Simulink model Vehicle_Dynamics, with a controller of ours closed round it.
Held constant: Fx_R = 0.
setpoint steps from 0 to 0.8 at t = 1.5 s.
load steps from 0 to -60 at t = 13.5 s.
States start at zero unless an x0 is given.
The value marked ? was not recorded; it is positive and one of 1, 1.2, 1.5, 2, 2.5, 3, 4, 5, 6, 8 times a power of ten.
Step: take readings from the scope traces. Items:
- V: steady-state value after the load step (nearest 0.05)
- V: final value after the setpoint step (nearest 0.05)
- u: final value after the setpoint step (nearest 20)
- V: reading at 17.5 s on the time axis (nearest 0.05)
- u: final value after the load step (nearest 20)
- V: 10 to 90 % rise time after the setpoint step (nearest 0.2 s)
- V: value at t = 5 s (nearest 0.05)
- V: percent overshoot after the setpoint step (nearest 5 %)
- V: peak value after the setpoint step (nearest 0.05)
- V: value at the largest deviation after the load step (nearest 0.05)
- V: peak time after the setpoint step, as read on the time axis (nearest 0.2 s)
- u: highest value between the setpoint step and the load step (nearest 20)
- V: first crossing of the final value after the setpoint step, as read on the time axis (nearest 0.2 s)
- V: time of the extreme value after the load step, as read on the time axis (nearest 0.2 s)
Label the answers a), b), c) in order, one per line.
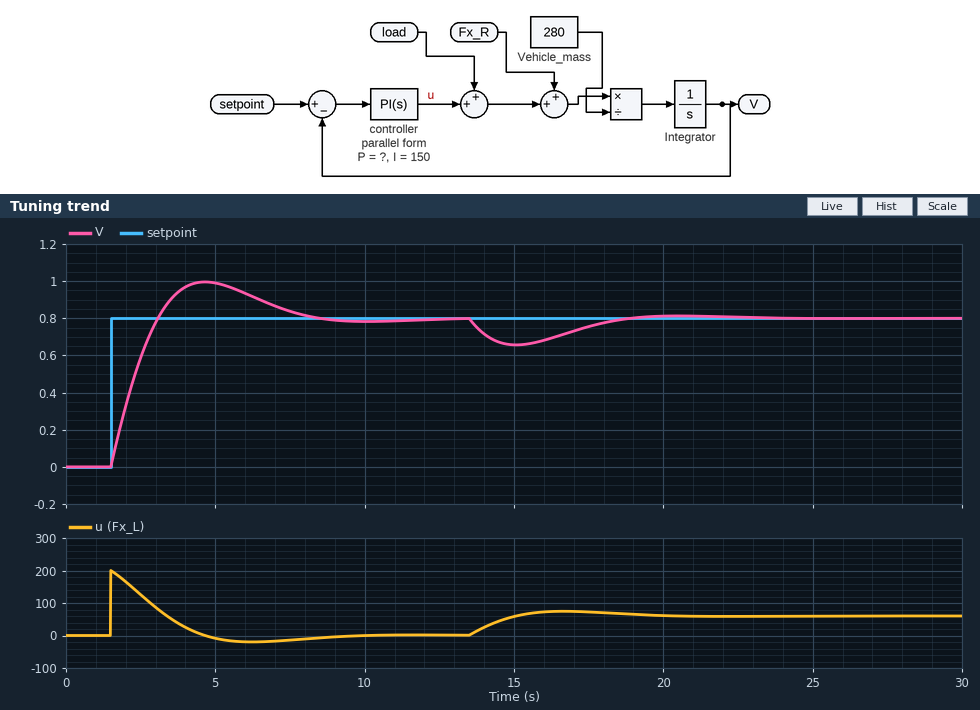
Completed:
a) 0.80
b) 0.80
c) 0
d) 0.75
e) 60
f) 1.2 s
g) 1.00
h) 25 %
i) 1.00
j) 0.65
k) 4.6 s
l) 200
m) 3.0 s
n) 15.0 s
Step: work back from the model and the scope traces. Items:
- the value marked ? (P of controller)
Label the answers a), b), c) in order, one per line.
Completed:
a) 250
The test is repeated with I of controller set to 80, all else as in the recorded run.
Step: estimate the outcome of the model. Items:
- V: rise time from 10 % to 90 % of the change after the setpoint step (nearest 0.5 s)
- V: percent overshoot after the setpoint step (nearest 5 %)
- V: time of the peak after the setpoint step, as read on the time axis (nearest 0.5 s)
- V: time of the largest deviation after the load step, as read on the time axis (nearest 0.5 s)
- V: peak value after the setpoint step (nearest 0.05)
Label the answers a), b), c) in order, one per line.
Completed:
a) 1.5 s
b) 15 %
c) 5.5 s
d) 15.5 s
e) 0.95
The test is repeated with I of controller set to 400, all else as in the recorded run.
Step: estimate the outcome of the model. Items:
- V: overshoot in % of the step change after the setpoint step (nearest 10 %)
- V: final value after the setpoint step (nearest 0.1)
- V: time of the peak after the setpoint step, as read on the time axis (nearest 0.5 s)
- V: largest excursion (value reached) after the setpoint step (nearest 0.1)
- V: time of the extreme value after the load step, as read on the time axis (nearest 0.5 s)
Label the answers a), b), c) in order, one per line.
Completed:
a) 40 %
b) 0.8
c) 3.5 s
d) 1.1
e) 14.5 s
